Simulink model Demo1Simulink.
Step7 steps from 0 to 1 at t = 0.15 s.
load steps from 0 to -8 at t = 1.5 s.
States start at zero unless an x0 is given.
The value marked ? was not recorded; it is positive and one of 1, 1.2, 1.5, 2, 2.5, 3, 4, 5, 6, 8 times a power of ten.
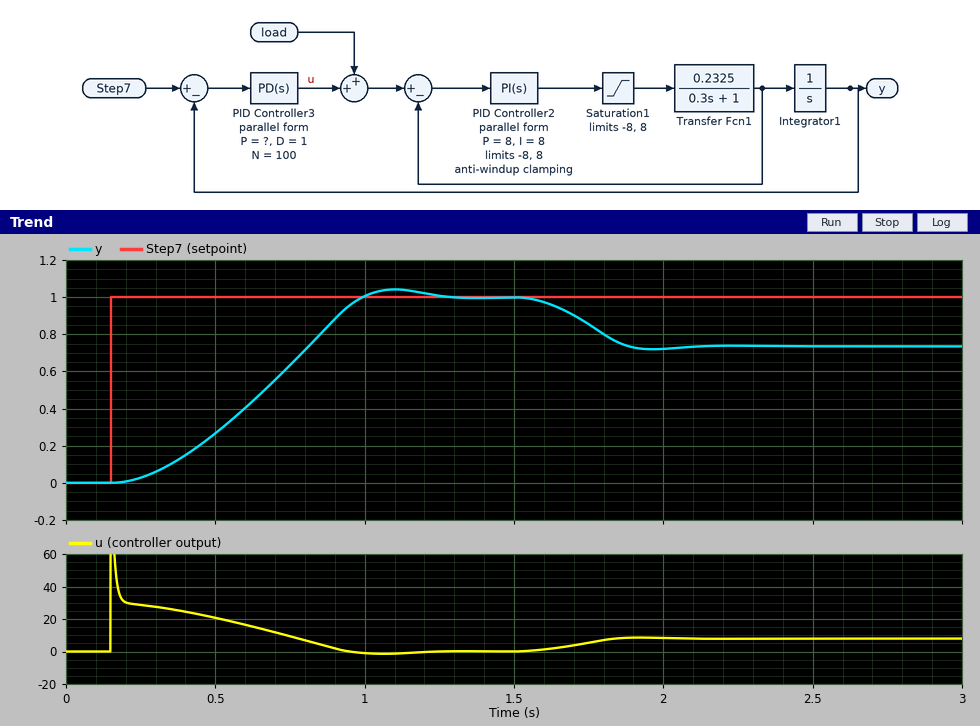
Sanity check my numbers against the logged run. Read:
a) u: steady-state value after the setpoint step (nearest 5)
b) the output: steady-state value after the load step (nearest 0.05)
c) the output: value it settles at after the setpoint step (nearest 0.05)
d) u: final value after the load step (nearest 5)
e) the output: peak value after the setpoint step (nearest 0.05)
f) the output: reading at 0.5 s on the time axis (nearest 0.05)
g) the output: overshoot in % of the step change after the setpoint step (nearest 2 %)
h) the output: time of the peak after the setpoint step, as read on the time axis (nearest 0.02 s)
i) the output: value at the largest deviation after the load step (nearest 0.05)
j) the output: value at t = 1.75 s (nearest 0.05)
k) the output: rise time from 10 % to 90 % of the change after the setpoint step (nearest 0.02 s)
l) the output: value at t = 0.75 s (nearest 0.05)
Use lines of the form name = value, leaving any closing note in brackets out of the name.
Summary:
u: steady-state value after the setpoint step = 0
the output: steady-state value after the load step = 0.75
the output: value it settles at after the setpoint step = 1.00
u: final value after the load step = 10
the output: peak value after the setpoint step = 1.05
the output: reading at 0.5 s on the time axis = 0.25
the output: overshoot in % of the step change after the setpoint step = 4 %
the output: time of the peak after the setpoint step, as read on the time axis = 1.10 s
the output: value at the largest deviation after the load step = 0.70
the output: value at t = 1.75 s = 0.85
the output: rise time from 10 % to 90 % of the change after the setpoint step = 0.56 s
the output: value at t = 0.75 s = 0.65
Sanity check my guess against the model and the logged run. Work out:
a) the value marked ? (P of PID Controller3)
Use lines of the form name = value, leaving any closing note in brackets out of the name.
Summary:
the value marked ? = 30
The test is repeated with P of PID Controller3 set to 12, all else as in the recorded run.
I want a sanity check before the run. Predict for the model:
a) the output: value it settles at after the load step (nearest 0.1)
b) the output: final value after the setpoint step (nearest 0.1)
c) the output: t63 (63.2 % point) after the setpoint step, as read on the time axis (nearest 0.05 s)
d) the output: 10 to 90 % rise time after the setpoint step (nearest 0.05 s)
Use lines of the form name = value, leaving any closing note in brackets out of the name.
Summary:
the output: value it settles at after the load step = 0.3
the output: final value after the setpoint step = 1.0
the output: t63 (63.2 % point) after the setpoint step, as read on the time axis = 0.75 s
the output: 10 to 90 % rise time after the setpoint step = 0.60 s
